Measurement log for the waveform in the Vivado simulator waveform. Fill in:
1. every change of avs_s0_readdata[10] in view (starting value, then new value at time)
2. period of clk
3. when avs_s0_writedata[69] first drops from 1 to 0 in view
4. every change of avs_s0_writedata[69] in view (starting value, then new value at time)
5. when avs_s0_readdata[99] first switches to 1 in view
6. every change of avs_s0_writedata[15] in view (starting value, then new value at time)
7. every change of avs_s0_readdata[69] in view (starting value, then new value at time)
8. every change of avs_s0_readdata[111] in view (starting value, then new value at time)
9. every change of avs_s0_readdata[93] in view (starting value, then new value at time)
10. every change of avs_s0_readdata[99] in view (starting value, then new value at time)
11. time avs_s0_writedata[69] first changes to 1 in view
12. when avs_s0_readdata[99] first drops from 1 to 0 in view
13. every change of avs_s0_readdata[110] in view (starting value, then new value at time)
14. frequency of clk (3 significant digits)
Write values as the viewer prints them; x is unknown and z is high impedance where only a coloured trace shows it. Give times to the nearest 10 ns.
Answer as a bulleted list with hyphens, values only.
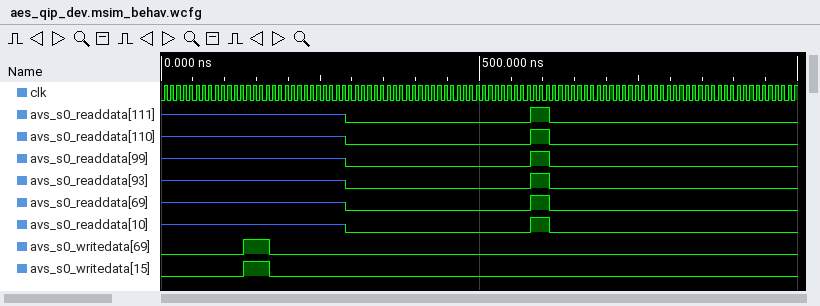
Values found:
- z, 0 at 290 ns, 1 at 580 ns, 0 at 610 ns
- 10 ns
- 170 ns
- 0, 1 at 130 ns, 0 at 170 ns
- 580 ns
- 0, 1 at 130 ns, 0 at 170 ns
- z, 0 at 290 ns, 1 at 580 ns, 0 at 610 ns
- z, 0 at 290 ns, 1 at 580 ns, 0 at 610 ns
- z, 0 at 290 ns, 1 at 580 ns, 0 at 610 ns
- z, 0 at 290 ns, 1 at 580 ns, 0 at 610 ns
- 130 ns
- 610 ns
- z, 0 at 290 ns, 1 at 580 ns, 0 at 610 ns
- 100 MHz
